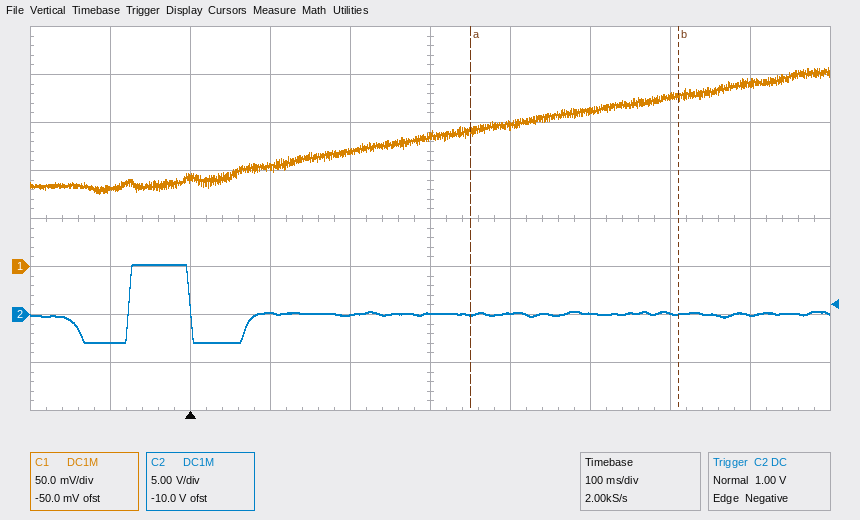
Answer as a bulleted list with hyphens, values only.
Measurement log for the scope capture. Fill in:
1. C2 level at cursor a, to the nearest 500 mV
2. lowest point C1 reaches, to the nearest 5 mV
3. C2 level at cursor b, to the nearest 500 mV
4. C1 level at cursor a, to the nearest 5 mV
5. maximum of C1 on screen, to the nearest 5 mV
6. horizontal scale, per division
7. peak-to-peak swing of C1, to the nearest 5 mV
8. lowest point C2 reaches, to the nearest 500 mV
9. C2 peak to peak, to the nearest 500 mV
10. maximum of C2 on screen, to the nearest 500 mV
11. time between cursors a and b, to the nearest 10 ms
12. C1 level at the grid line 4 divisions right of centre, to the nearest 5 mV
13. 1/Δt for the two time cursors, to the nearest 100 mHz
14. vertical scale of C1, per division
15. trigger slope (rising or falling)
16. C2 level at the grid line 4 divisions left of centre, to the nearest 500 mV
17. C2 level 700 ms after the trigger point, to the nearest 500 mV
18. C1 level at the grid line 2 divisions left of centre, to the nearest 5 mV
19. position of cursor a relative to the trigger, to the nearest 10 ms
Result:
- 0.0 V
- 75 mV
- 0.0 V
- 140 mV
- 205 mV
- 100 ms
- 130 mV
- -3.0 V
- 8.0 V
- 5.0 V
- 260 ms
- 190 mV
- 3.8 Hz
- 50 mV
- falling
- -3.0 V
- 0.0 V
- 105 mV
- +350 ms
